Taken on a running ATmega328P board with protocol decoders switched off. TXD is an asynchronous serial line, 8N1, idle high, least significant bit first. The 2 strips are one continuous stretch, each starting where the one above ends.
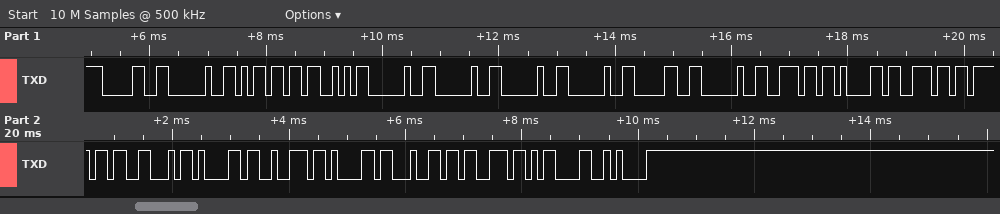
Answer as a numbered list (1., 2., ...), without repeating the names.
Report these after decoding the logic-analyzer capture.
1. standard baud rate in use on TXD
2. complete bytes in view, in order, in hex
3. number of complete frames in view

1. 9600 baud
2. 30 20 6D 53 20 20 20 20 30 20 6E 61 6E 6F 46 61 72 61 64 73 0D 0A
3. 22
